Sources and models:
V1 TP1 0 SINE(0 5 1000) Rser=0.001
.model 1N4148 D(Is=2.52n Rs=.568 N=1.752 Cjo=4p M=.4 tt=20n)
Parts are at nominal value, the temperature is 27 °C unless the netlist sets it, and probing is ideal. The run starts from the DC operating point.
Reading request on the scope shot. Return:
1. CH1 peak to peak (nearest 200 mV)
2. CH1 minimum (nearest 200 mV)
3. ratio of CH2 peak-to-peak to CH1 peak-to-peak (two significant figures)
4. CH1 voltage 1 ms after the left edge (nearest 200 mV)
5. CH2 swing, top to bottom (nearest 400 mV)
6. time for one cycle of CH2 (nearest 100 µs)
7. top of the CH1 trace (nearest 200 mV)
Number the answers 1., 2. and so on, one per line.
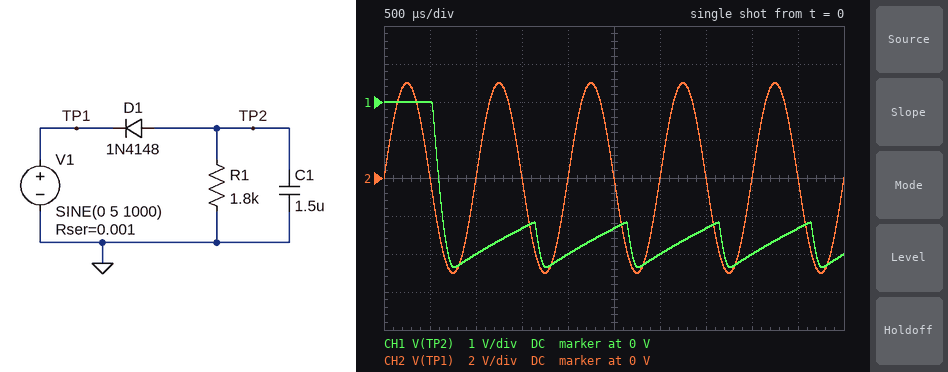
1. 4.4 V
2. -4.4 V
3. 2.3
4. -4.0 V
5. 10.0 V
6. 1.0 ms
7. 0 V
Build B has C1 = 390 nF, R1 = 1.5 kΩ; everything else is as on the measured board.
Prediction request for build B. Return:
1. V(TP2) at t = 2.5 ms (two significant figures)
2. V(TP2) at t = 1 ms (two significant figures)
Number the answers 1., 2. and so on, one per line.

1. -1.3 V
2. -3.0 V
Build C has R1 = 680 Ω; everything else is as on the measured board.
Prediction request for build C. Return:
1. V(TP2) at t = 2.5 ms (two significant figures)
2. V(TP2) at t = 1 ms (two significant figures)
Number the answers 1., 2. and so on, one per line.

1. -2.1 V
2. -3.5 V
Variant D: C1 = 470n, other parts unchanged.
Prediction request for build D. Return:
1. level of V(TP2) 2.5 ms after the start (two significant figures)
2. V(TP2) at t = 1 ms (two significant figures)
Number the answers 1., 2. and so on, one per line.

1. -1.9 V
2. -3.4 V
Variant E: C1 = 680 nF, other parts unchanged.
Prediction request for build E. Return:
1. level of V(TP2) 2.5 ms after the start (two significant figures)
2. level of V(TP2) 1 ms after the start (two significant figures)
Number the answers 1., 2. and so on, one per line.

1. -2.4 V
2. -3.6 V
